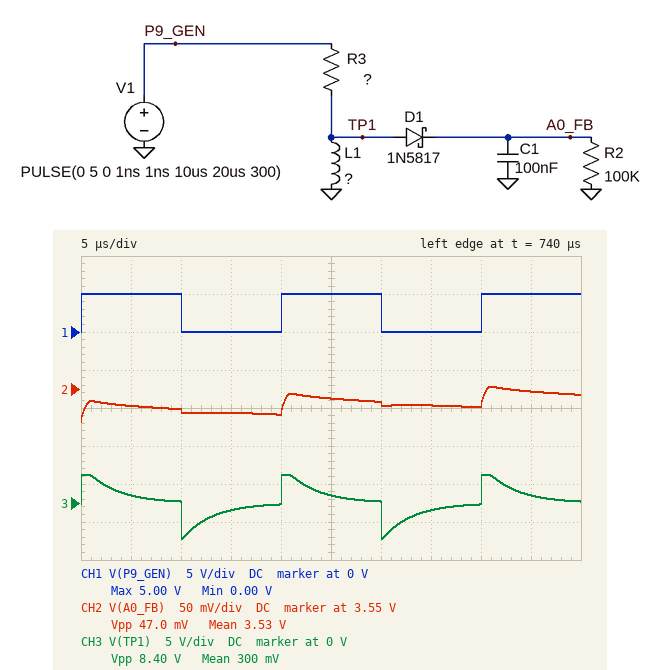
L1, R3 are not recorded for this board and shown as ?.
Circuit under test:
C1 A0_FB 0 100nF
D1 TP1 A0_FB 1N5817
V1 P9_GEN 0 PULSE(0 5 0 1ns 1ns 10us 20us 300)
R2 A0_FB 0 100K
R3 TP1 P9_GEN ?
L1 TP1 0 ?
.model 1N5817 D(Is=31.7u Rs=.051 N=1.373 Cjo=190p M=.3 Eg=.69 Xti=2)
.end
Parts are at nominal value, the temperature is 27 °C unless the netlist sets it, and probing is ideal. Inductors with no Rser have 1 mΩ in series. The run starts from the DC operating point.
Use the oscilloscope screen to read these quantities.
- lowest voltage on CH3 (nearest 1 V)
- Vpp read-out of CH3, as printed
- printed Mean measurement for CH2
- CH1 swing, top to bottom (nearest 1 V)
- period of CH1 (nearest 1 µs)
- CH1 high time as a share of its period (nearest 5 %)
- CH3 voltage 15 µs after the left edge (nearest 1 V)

-5 V
8.40 V
3.53 V
5 V
20 µs
50 %
-1 V
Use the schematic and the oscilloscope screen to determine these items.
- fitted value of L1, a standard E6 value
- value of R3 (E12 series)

680 µH
220 Ω
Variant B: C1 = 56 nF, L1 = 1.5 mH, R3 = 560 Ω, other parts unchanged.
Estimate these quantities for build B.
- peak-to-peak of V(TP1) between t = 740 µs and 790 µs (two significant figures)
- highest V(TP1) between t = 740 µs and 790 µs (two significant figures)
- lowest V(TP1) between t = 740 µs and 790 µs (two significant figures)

7.9 V
3.3 V
-4.6 V
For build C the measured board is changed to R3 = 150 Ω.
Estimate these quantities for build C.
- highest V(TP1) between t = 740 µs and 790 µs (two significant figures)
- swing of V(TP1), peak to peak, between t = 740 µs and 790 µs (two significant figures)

3.8 V
8.3 V
